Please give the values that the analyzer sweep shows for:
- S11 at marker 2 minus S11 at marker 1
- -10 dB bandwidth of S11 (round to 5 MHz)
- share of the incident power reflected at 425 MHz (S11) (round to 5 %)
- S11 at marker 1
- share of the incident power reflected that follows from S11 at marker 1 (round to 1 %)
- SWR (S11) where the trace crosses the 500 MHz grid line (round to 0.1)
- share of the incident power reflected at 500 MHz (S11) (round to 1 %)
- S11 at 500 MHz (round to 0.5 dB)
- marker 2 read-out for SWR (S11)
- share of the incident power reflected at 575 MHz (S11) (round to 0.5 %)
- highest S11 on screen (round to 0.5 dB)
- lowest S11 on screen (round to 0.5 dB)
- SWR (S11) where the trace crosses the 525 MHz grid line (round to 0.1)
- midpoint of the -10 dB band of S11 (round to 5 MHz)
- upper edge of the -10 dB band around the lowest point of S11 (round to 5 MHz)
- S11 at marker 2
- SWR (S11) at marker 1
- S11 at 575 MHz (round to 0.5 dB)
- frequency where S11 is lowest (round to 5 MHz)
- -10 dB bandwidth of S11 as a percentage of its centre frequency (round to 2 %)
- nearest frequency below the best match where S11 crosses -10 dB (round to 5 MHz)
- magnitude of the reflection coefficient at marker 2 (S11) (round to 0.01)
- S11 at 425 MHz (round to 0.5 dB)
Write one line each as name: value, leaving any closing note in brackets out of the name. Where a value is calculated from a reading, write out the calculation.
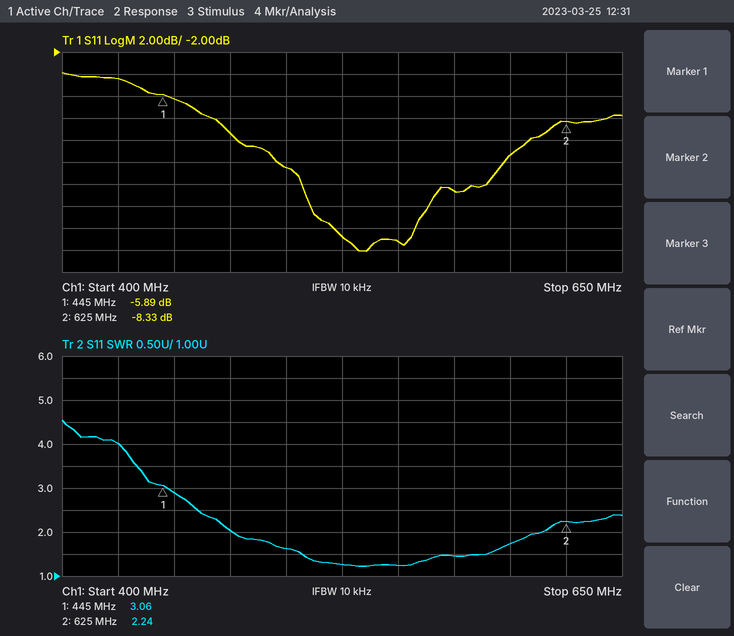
S11 at marker 2 minus S11 at marker 1: -8.33 − (-5.89) = -2.44 dB
-10 dB bandwidth of S11: 610 MHz − 480 MHz = 130 MHz
share of the incident power reflected at 425 MHz (S11): 10^(-4.5/10) ≈ 35 %
S11 at marker 1: -5.89 dB
share of the incident power reflected that follows from S11 at marker 1: 10^(-5.89/10) ≈ 26 %
SWR (S11) where the trace crosses the 500 MHz grid line: 1.6
share of the incident power reflected at 500 MHz (S11): 10^(-12.5/10) ≈ 6 %
S11 at 500 MHz: -12.5 dB
marker 2 read-out for SWR: 2.24
share of the incident power reflected at 575 MHz (S11): 10^(-14.5/10) ≈ 3.5 %
highest S11 on screen: -4.0 dB
lowest S11 on screen: -20.0 dB
SWR (S11) where the trace crosses the 525 MHz grid line: 1.3
midpoint of the -10 dB band of S11: 545 MHz
upper edge of the -10 dB band around the lowest point of S11: 610 MHz
S11 at marker 2: -8.33 dB
SWR (S11) at marker 1: 3.06
S11 at 575 MHz: -14.5 dB
frequency where S11 is lowest: 535 MHz
-10 dB bandwidth of S11 as a percentage of its centre frequency: 130 MHz / 545 MHz ≈ 24 %
nearest frequency below the best match where S11 crosses -10 dB: 480 MHz
magnitude of the reflection coefficient at marker 2 (S11): 10^(-8.33/20) ≈ 0.38
S11 at 425 MHz: -4.5 dB
